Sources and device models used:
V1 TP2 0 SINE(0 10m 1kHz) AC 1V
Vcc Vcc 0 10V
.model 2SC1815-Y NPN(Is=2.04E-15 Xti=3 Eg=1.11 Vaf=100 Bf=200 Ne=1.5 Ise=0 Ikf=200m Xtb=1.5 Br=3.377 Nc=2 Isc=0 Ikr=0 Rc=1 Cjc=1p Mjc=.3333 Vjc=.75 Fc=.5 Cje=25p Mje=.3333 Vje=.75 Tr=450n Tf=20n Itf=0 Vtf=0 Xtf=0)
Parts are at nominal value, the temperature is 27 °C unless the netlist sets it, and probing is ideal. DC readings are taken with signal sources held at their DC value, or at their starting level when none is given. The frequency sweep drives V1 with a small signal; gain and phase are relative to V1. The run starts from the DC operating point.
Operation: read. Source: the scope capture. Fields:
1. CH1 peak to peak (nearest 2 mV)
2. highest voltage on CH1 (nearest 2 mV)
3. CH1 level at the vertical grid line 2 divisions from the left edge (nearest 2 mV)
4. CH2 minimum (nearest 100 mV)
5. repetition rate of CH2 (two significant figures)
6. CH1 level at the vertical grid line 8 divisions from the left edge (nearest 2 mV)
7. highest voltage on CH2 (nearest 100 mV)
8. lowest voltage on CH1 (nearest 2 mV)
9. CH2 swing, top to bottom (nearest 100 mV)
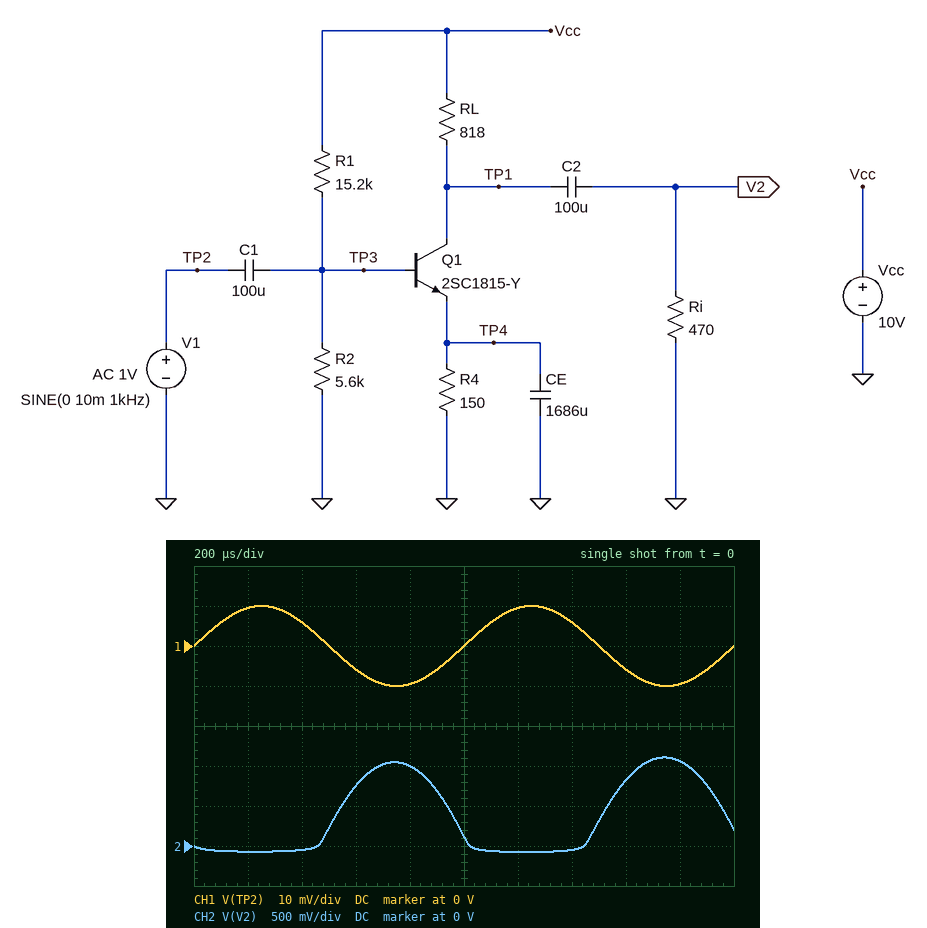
20 mV
10 mV
6 mV
-100 mV
1.0 kHz
-6 mV
1.1 V
-10 mV
1.2 V
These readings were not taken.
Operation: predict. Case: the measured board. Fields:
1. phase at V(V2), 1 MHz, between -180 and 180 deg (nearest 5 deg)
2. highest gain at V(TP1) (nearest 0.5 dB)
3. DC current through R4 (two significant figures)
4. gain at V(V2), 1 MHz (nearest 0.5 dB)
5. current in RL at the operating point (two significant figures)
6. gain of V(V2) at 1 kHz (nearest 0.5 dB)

120 deg
31.5 dB
10 mA
26.5 dB
10 mA
31.5 dB
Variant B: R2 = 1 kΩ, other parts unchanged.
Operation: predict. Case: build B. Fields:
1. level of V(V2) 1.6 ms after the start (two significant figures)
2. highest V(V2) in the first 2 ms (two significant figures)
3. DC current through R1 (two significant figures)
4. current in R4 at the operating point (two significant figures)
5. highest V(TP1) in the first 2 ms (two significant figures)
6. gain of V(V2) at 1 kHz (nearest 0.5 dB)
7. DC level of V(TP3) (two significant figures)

2.5 mV
3.9 mV
620 µA
41 µA
10 V
-6.5 dB
620 mV
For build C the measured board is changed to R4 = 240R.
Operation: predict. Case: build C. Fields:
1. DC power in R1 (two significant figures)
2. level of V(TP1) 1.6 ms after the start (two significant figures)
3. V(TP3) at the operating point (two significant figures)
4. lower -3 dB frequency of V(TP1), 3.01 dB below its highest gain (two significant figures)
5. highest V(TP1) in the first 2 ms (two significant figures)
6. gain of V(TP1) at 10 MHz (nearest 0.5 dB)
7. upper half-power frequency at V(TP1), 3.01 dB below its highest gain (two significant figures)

3.7 mW
4.4 V
2.5 V
28 Hz
4.6 V
38.0 dB
770 MHz
